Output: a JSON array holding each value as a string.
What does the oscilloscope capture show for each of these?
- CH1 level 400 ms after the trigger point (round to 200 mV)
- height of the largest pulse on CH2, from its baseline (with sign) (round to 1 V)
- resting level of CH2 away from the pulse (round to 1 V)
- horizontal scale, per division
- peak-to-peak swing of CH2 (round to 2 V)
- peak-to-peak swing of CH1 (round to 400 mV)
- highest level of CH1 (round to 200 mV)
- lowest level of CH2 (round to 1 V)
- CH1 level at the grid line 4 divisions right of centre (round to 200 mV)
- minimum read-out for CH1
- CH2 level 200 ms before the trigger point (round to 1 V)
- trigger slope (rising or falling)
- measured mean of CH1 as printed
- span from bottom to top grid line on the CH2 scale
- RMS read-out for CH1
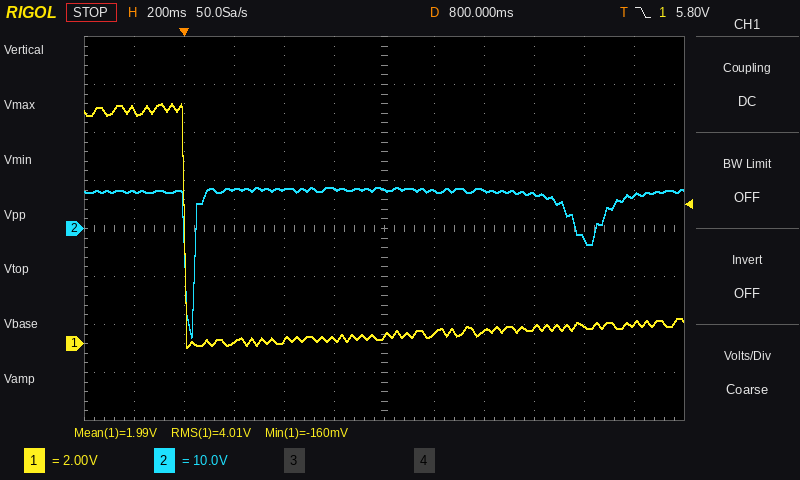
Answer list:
["200 mV", "-31 V", "8 V", "200 ms", "32 V", "10.0 V", "10.0 V", "-23 V", "800 mV", "-160 mV", "8 V", "falling", "1.99 V", "80 V", "4.01 V"]
